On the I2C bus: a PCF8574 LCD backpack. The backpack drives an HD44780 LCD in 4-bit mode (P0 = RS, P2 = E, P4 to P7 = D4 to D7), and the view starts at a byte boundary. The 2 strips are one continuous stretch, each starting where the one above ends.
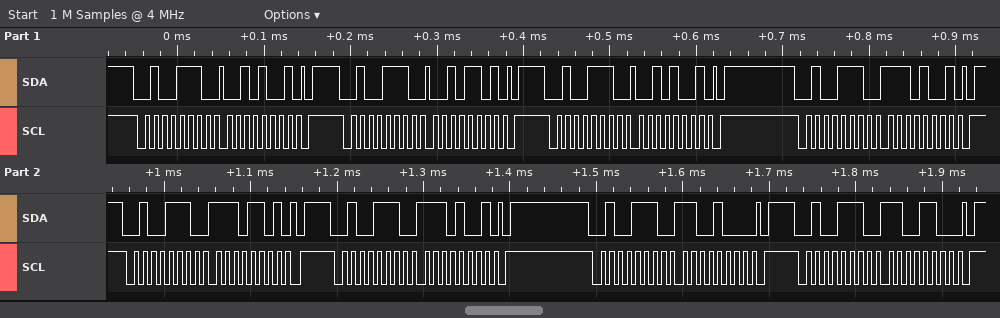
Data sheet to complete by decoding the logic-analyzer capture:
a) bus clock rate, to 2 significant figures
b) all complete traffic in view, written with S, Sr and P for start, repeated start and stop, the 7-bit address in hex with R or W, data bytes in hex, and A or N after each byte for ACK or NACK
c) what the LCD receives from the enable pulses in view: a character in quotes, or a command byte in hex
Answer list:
100 kHz
S 27W A 29 A P S 27W A 2D A P S 27W A 29 A P S 27W A E9 A P S 27W A ED A P S 27W A E9 A P S 27W A C8 A P S 27W A CC A P
'.'
